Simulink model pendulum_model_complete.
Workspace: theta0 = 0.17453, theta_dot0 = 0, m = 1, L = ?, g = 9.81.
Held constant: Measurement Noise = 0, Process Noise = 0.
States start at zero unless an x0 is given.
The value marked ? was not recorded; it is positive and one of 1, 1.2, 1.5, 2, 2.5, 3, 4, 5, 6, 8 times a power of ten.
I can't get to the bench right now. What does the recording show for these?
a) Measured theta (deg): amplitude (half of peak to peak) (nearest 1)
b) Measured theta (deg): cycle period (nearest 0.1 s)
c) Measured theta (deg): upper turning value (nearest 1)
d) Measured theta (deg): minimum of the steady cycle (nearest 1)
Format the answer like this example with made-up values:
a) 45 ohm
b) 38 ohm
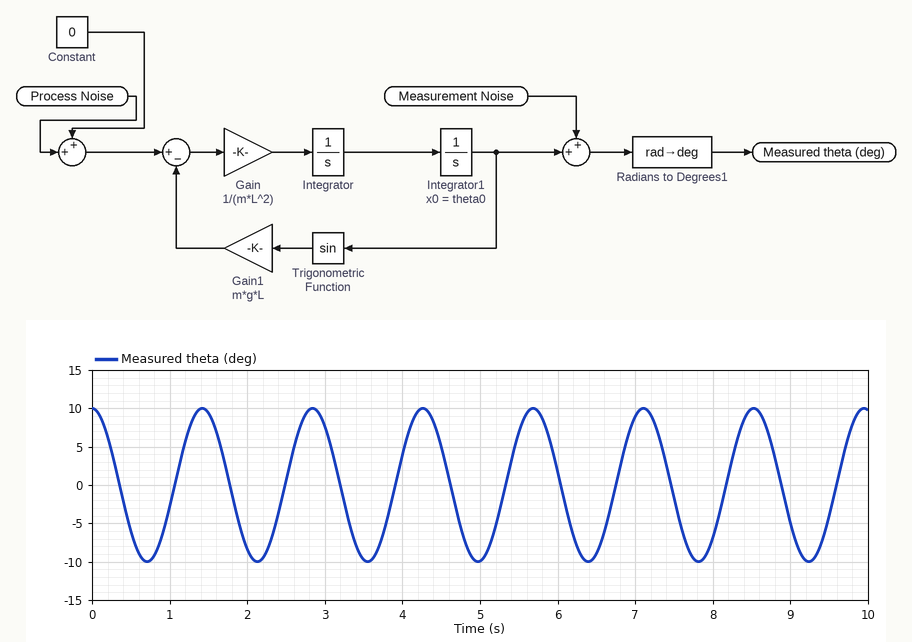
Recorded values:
a) 10
b) 1.4 s
c) 10
d) -10
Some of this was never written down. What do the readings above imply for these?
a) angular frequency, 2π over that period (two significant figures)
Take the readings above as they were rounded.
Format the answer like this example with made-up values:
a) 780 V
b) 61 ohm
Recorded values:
a) 4.5 rad/s
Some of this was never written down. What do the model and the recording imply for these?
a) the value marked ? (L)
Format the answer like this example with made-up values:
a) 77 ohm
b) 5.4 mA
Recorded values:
a) 0.5
